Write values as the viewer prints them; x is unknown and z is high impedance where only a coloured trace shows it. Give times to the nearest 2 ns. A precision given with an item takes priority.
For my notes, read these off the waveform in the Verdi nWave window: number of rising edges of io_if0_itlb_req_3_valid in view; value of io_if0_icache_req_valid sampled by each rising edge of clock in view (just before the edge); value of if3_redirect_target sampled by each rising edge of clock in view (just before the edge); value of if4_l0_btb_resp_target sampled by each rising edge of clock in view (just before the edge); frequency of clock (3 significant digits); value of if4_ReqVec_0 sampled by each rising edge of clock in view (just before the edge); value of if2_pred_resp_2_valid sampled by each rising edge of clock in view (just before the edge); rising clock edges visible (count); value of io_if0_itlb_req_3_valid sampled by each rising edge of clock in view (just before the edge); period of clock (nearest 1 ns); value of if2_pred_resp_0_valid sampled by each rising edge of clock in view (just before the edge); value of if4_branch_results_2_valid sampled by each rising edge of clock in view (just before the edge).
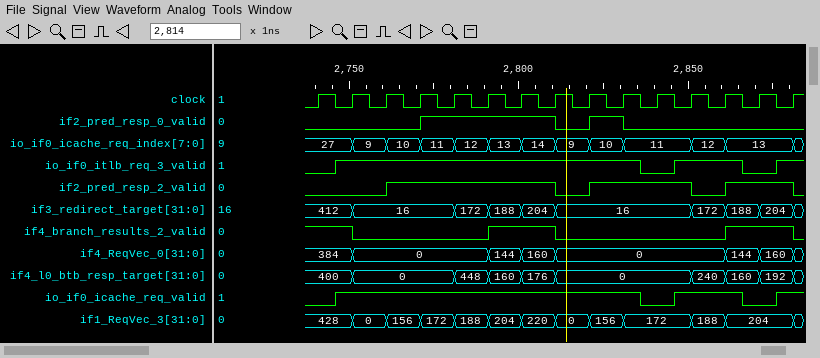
3
0 1 1 1 1 1 1 1 1 1 0 1 1 0 1
412, 412, 16, 16, 16, 172, 188, 204, 16, 16, 16, 16, 172, 188, 204
400, 400, 0, 0, 0, 448, 160, 176, 0, 0, 0, 0, 240, 160, 192
100 MHz
384, 384, 0, 0, 0, 0, 144, 160, 0, 0, 0, 0, 0, 144, 160
0 0 0 1 1 1 1 1 0 1 1 1 0 1 1
15
0 1 1 1 1 1 1 1 1 1 0 1 1 0 1
10 ns
0 0 0 0 1 1 1 1 0 1 0 0 0 0 0
1 1 0 0 0 0 1 1 0 0 0 0 0 1 1
